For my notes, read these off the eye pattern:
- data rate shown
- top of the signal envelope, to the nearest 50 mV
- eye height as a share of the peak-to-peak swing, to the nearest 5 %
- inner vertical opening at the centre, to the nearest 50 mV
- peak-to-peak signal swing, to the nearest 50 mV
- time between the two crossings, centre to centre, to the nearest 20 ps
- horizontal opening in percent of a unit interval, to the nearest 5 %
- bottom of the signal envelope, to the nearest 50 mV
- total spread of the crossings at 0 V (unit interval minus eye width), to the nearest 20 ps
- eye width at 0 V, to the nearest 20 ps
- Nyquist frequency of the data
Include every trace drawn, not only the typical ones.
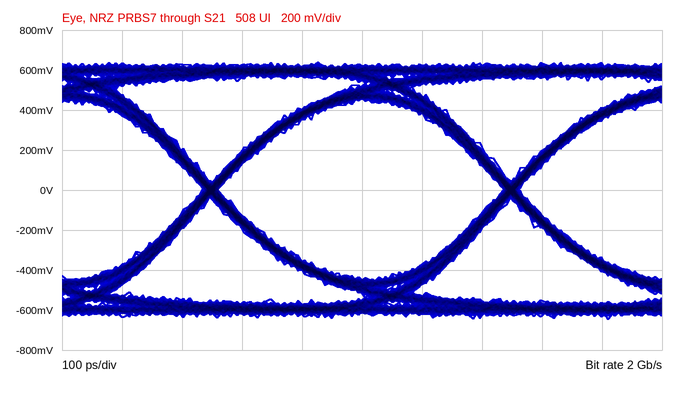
2 Gb/s
650 mV
70 %
900 mV
1.30 V
500 ps
95 %
-650 mV
20 ps
480 ps
1 GHz
